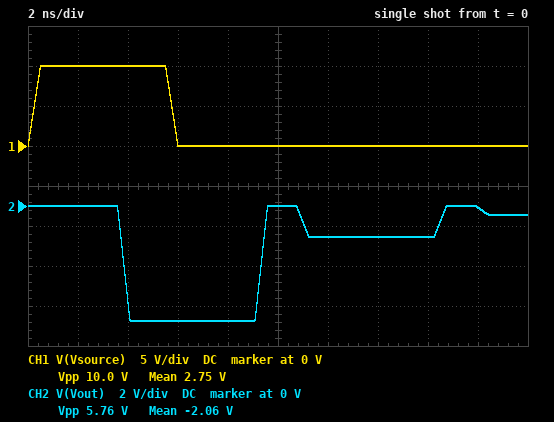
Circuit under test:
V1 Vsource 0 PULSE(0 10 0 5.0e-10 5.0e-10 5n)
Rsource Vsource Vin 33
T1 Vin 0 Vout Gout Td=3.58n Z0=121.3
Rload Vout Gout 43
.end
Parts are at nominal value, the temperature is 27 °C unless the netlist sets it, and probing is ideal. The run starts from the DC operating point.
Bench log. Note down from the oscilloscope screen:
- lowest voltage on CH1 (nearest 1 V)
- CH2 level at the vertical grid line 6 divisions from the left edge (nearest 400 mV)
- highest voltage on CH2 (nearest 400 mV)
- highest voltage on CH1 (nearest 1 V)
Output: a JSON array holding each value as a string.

["0 V", "-1.6 V", "0 V", "10 V"]
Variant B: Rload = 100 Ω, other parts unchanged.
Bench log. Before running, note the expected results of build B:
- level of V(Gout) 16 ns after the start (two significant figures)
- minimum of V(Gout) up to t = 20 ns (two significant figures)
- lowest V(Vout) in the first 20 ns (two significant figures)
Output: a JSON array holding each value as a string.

["-630 mV", "-11 V", "-4.3 V"]
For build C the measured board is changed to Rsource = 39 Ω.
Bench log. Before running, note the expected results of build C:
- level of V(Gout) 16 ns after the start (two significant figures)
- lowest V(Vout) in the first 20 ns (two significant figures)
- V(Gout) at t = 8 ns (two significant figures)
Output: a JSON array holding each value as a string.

["-2.3 V", "-5.5 V", "-9.5 V"]
